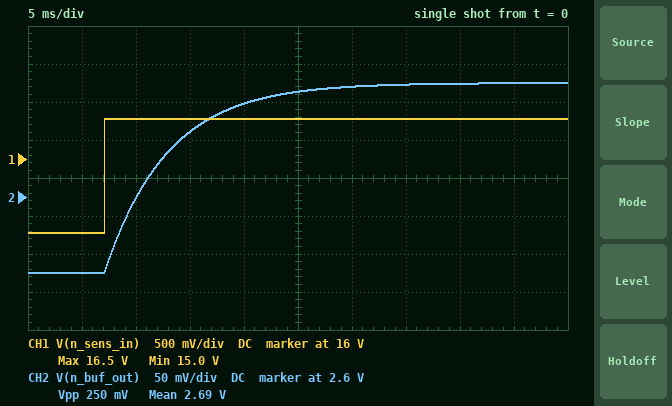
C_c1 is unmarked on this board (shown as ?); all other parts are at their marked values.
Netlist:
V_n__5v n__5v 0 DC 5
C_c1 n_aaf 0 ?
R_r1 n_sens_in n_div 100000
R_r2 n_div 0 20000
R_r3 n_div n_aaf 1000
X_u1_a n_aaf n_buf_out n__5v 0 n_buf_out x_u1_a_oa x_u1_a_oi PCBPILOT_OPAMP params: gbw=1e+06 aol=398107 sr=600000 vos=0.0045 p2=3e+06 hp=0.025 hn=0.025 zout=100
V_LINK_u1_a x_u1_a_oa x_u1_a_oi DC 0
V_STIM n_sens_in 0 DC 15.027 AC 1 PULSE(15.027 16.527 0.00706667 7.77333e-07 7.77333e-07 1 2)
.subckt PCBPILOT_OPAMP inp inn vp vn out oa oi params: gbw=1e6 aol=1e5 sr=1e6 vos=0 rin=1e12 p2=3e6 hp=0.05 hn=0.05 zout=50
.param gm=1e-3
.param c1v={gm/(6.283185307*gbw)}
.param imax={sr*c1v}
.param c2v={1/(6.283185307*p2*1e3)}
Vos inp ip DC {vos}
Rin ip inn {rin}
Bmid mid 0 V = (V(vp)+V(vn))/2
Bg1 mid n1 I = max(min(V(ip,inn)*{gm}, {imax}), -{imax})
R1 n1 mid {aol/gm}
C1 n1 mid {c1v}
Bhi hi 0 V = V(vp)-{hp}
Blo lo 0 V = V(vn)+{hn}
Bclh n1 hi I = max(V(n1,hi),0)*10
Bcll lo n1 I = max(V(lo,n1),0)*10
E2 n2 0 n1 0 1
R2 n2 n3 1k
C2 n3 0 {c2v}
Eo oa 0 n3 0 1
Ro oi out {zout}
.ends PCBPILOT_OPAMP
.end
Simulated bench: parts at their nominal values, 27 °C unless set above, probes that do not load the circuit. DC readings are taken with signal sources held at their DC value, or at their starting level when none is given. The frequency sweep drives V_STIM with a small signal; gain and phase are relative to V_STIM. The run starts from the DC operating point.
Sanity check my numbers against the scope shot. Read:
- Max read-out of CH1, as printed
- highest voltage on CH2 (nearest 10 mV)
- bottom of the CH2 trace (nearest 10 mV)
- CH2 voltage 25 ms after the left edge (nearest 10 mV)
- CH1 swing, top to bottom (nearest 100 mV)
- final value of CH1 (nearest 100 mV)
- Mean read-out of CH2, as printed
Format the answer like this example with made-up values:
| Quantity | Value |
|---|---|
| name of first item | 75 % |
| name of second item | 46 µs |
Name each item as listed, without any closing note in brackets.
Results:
| Quantity | Value |
|---|---|
| Max read-out of CH1, as printed | 16.5 V |
| highest voltage on CH2 | 2.75 V |
| bottom of the CH2 trace | 2.50 V |
| CH2 voltage 25 ms after the left edge | 2.74 V |
| CH1 swing, top to bottom | 1.5 V |
| final value of CH1 | 16.5 V |
| Mean read-out of CH2, as printed | 2.69 V |
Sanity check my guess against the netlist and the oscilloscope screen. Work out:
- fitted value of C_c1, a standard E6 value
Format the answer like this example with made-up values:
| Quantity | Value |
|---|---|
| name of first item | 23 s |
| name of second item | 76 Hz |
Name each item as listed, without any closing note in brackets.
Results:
| Quantity | Value |
|---|---|
| fitted value of C_c1, a standard E6 value | 330 nF |
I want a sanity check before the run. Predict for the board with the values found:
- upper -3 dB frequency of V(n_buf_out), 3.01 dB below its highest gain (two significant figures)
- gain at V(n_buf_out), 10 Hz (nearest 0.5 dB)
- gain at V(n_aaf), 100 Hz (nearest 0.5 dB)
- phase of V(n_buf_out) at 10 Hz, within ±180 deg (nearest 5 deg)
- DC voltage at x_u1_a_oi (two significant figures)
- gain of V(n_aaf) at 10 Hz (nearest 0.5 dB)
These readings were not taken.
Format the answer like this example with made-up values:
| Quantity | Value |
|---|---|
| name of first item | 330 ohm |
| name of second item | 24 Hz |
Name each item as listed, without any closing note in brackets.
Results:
| Quantity | Value |
|---|---|
| upper -3 dB frequency of V(n_buf_out), 3.01 dB below its highest gain | 27 Hz |
| gain at V(n_buf_out), 10 Hz | -16.0 dB |
| gain at V(n_aaf), 100 Hz | -27.0 dB |
| phase of V(n_buf_out) at 10 Hz, within ±180 deg | -20 deg |
| DC voltage at x_u1_a_oi | 2.5 V |
| gain of V(n_aaf) at 10 Hz | -16.0 dB |
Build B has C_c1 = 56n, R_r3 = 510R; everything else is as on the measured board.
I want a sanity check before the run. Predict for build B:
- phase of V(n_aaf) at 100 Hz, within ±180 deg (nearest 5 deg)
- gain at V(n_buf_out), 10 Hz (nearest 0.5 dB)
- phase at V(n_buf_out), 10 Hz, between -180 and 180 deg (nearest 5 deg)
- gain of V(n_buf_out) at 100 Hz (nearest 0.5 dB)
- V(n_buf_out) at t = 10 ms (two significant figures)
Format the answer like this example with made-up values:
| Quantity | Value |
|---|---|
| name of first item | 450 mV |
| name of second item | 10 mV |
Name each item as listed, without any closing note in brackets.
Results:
| Quantity | Value |
|---|---|
| phase of V(n_aaf) at 100 Hz, within ±180 deg | -30 deg |
| gain at V(n_buf_out), 10 Hz | -15.5 dB |
| phase at V(n_buf_out), 10 Hz, between -180 and 180 deg | -5 deg |
| gain of V(n_buf_out) at 100 Hz | -17.0 dB |
| V(n_buf_out) at t = 10 ms | 2.7 V |
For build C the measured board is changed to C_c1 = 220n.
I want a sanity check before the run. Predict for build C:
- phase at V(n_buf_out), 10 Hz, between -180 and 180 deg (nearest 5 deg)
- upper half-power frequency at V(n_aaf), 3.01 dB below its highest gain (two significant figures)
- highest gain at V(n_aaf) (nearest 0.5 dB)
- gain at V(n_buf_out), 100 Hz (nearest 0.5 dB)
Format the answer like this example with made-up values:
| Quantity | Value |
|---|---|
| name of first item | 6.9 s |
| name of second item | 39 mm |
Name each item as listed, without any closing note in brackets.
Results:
| Quantity | Value |
|---|---|
| phase at V(n_buf_out), 10 Hz, between -180 and 180 deg | -15 deg |
| upper half-power frequency at V(n_aaf), 3.01 dB below its highest gain | 41 Hz |
| highest gain at V(n_aaf) | -15.5 dB |
| gain at V(n_buf_out), 100 Hz | -24.0 dB |
